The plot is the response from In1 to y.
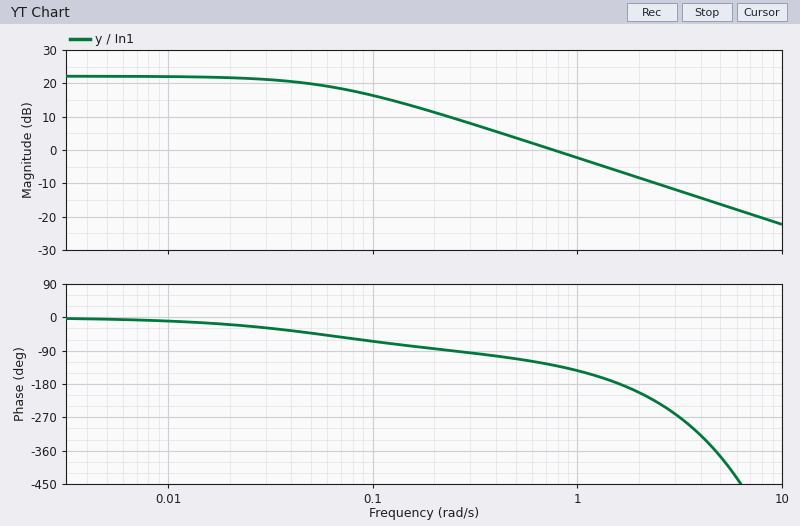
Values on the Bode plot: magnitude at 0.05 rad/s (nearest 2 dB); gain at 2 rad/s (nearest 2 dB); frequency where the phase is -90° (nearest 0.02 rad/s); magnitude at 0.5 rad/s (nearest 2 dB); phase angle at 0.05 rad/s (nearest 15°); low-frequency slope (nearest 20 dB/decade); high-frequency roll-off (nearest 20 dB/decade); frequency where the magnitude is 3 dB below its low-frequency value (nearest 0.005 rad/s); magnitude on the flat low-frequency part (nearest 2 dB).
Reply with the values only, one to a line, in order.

20 dB
-8 dB
0.24 rad/s
4 dB
-45°
0 dB/decade
-20 dB/decade
0.060 rad/s
22 dB
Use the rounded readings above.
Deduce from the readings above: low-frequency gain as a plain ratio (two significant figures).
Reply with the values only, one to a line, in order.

13
